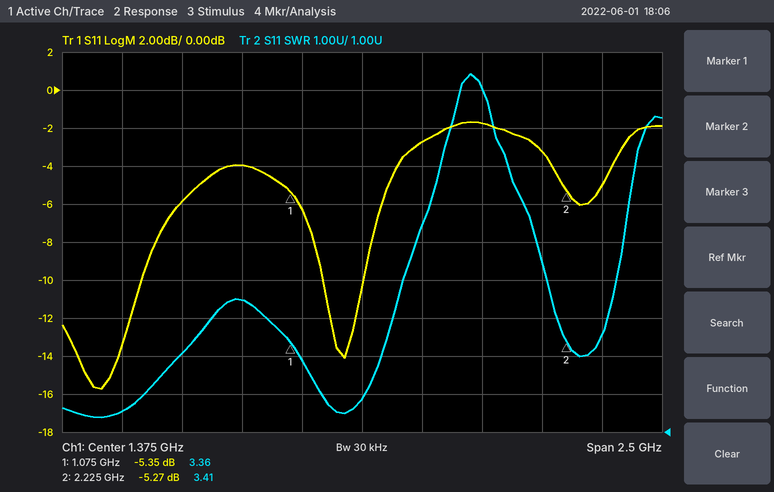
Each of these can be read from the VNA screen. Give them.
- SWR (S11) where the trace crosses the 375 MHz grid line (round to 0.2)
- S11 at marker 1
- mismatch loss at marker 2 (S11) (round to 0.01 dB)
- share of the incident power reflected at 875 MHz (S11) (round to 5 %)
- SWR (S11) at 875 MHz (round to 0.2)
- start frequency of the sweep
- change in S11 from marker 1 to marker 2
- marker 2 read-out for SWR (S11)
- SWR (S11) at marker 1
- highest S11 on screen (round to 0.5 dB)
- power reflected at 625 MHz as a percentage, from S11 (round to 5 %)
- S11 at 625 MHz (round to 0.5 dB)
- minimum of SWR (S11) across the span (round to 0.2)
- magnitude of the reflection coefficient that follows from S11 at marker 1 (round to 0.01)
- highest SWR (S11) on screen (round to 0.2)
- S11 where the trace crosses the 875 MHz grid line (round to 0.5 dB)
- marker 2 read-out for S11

1.6
-5.35 dB
1.53 dB
40 %
4.4
125 MHz
0.08 dB
3.41
3.36
-1.5 dB
25 %
-6.0 dB
1.4
0.54
10.4
-4.0 dB
-5.27 dB
